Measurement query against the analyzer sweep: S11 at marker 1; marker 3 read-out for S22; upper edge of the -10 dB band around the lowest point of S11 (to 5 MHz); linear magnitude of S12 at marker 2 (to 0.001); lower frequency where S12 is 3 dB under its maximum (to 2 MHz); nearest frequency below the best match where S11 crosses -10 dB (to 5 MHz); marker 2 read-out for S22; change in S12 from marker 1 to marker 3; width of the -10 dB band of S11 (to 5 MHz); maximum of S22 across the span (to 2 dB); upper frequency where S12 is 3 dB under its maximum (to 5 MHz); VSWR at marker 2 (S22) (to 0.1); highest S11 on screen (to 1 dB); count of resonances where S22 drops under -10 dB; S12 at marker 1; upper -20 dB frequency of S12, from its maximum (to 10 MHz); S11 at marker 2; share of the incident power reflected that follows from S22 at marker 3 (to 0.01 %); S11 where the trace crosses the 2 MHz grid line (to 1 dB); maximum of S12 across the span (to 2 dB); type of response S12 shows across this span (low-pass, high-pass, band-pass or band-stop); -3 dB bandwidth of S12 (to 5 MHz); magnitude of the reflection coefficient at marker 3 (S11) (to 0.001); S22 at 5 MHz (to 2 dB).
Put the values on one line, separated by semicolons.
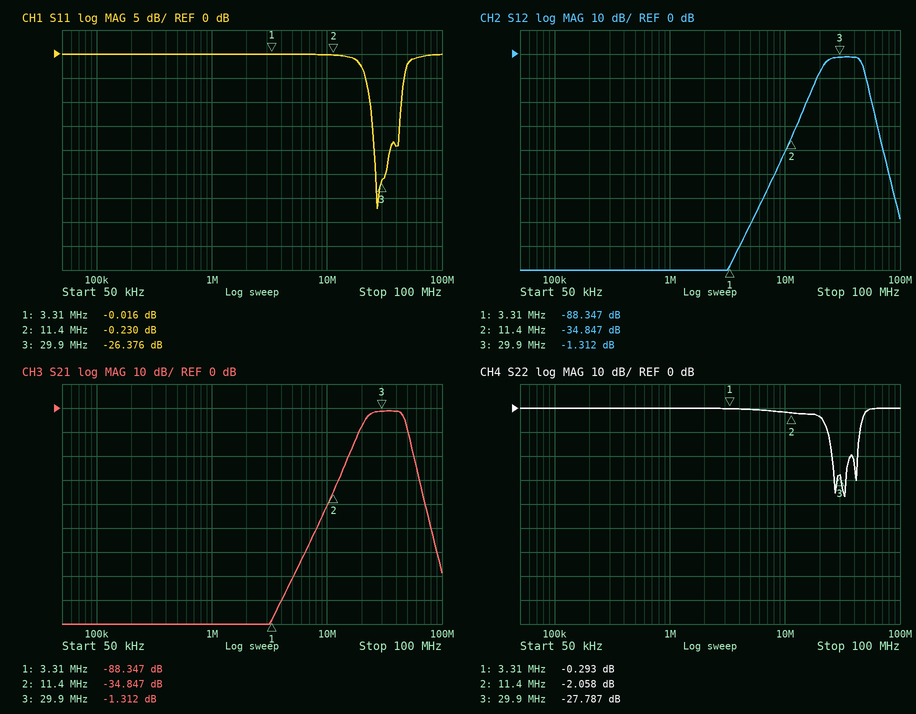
-0.016 dB; -27.787 dB; 45 MHz; 0.018; 22 MHz; 25 MHz; -2.058 dB; 87.035 dB; 20 MHz; 0 dB; 45 MHz; 8.5; 0 dB; 3; -88.347 dB; 60 MHz; -0.230 dB; 0.17 %; 0 dB; -2 dB; band-pass; 25 MHz; 0.048; 0 dB
